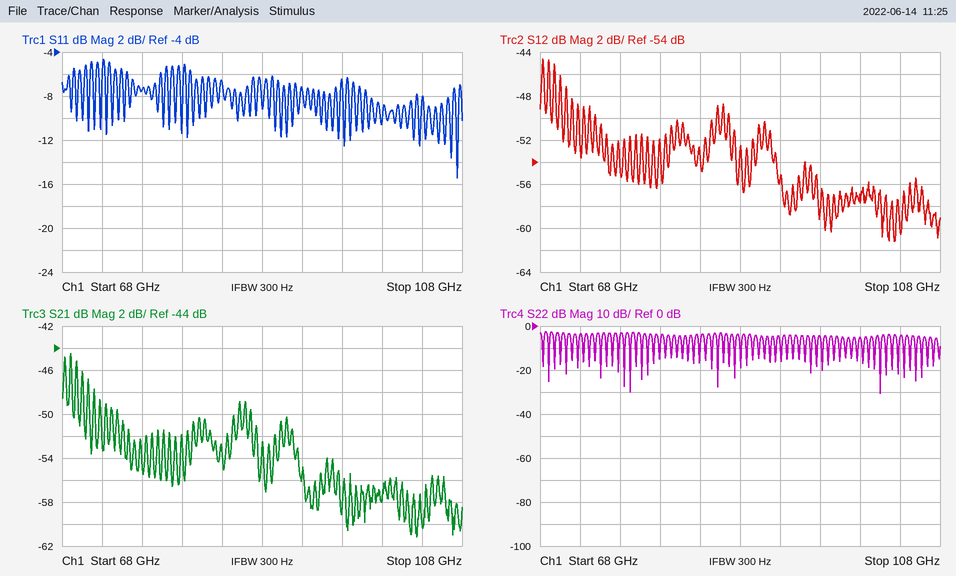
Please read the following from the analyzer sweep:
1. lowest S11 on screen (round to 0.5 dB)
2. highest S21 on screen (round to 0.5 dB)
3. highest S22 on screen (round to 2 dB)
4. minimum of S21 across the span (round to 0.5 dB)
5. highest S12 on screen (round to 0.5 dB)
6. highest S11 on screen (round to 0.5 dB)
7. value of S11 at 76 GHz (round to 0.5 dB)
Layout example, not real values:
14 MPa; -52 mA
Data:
-15.5 dB; -44.5 dB; -2 dB; -61.0 dB; -44.5 dB; -4.5 dB; -7.5 dB
